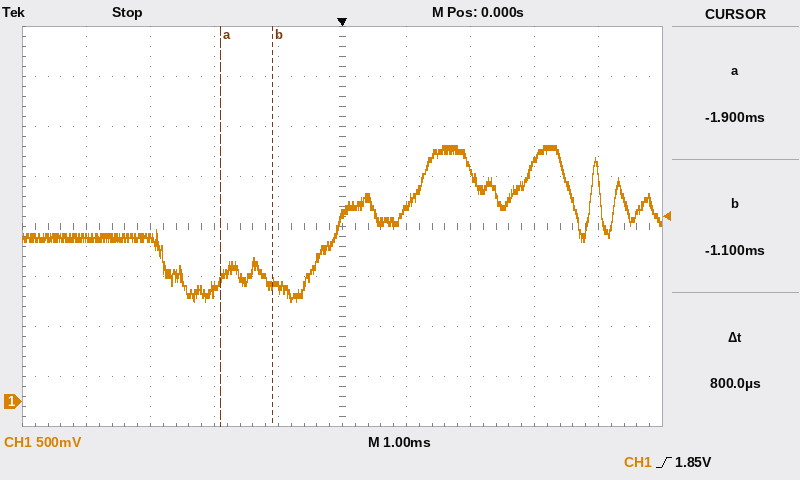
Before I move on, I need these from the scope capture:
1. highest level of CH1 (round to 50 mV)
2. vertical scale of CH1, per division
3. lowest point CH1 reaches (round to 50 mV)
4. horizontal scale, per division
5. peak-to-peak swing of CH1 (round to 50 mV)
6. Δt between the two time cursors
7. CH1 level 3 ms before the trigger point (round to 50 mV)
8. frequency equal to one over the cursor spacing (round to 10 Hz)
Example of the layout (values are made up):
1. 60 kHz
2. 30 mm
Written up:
1. 2.55 V
2. 500 mV
3. 1.00 V
4. 1 ms
5. 1.55 V
6. 800 µs
7. 1.65 V
8. 1.25 kHz
